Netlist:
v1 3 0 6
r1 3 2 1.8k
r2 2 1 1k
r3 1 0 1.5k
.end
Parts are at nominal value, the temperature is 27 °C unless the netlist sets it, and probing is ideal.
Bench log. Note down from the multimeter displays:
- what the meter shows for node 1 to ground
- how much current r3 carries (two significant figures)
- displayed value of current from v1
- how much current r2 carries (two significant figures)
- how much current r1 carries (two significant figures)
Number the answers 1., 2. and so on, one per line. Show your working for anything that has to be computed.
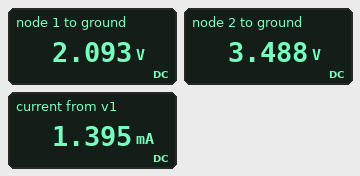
1. 2.093 V
2. (2.093 V) / 1.5 kΩ = 1.4 mA
3. 1.395 mA
4. (3.488 V - 2.093 V) / 1 kΩ = 1.4 mA
5. (6 V - 3.488 V) / 1.8 kΩ = 1.4 mA
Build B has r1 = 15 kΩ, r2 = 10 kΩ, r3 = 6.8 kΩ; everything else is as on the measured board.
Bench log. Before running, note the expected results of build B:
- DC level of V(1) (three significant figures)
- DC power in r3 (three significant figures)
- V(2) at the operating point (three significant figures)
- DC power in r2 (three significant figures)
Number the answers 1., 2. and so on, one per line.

1. 1.28 V
2. 242 µW
3. 3.17 V
4. 356 µW
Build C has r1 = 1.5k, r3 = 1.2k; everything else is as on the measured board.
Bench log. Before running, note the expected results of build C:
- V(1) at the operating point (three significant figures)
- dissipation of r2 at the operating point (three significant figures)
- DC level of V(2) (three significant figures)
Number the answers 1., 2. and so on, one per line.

1. 1.95 V
2. 2.63 mW
3. 3.57 V
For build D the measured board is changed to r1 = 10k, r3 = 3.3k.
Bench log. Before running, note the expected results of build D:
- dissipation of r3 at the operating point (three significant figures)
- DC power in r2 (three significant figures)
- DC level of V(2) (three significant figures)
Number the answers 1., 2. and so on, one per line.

1. 581 µW
2. 176 µW
3. 1.80 V
